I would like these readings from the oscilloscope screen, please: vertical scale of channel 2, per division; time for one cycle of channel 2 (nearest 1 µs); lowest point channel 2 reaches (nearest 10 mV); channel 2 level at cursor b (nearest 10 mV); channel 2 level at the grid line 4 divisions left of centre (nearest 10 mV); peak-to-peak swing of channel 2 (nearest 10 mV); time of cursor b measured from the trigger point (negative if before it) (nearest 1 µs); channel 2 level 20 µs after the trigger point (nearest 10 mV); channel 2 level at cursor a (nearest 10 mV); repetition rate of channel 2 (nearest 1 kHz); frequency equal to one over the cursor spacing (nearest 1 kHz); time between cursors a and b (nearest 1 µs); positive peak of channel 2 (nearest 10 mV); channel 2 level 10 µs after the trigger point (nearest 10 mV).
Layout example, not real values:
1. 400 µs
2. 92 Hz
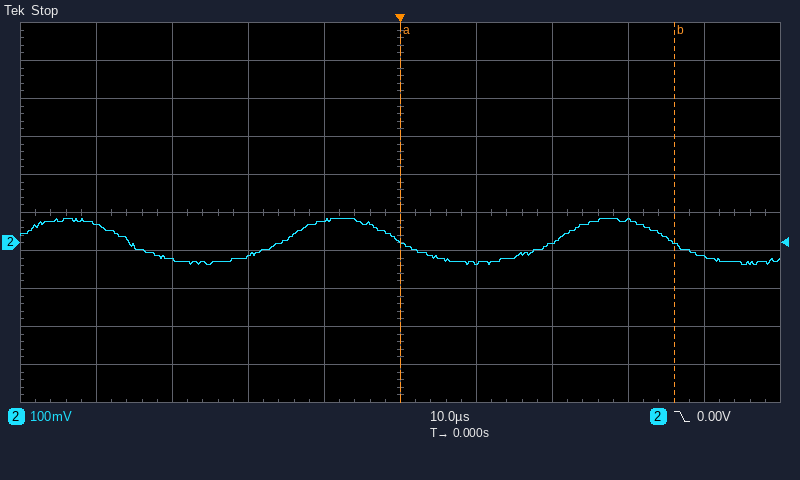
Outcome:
1. 100 mV
2. 36 µs
3. -60 mV
4. 0 mV
5. 50 mV
6. 120 mV
7. +36 µs
8. 0 mV
9. 0 mV
10. 28 kHz
11. 28 kHz
12. 36 µs
13. 60 mV
14. -50 mV
